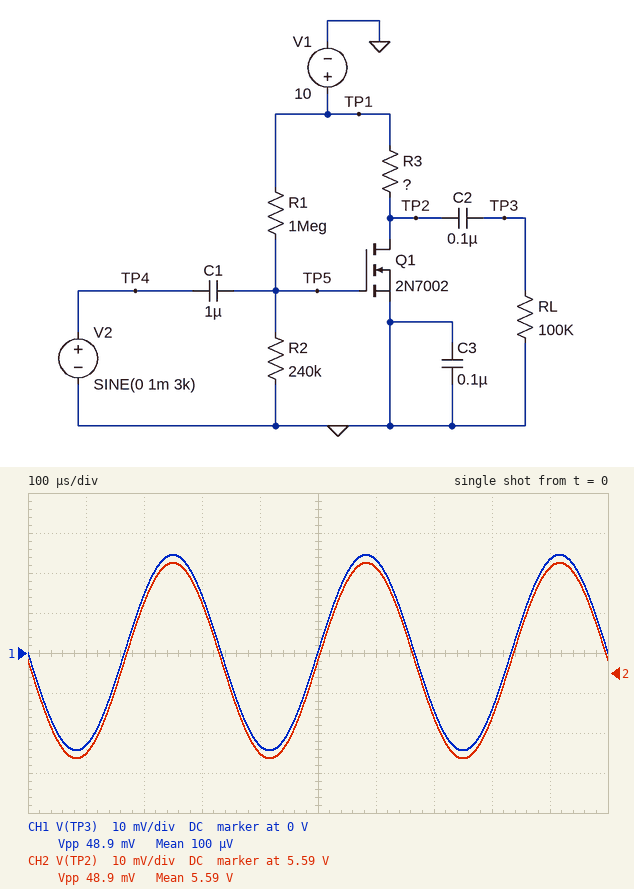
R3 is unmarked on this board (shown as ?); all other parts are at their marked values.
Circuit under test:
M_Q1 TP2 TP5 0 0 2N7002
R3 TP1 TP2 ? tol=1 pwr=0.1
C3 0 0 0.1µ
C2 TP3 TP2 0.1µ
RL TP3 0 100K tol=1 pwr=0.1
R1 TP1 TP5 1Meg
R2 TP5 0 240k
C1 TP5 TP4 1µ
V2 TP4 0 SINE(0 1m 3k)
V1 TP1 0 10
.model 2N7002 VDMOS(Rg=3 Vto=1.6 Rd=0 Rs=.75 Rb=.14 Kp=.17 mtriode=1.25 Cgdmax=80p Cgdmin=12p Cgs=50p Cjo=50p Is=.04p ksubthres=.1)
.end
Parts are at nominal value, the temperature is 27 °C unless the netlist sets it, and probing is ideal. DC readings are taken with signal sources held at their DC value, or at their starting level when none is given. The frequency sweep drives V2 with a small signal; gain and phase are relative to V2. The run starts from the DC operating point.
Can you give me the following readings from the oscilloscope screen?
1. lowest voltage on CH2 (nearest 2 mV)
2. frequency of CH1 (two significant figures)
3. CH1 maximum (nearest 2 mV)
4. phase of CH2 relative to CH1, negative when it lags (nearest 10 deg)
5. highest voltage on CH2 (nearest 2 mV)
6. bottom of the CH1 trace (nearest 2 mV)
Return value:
5.568 V
3.0 kHz
24 mV
0 deg
5.618 V
-24 mV
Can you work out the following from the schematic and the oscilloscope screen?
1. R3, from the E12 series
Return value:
470 Ω
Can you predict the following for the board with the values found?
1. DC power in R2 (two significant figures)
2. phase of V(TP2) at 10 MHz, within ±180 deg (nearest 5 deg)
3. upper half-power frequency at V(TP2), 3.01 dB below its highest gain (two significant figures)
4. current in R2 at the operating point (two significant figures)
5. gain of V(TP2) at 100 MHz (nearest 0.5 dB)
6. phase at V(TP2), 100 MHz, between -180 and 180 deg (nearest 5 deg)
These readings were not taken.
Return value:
16 µW
130 deg
8.5 MHz
8.1 µA
6.5 dB
75 deg
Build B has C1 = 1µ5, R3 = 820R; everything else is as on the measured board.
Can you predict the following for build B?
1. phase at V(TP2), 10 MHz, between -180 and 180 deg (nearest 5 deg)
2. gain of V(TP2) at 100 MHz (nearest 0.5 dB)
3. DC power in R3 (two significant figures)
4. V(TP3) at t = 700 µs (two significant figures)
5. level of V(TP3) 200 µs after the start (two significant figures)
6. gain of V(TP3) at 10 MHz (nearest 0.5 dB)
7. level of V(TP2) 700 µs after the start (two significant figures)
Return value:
100 deg
2.0 dB
72 mW
-25 mV
25 mV
20.5 dB
2.3 V
